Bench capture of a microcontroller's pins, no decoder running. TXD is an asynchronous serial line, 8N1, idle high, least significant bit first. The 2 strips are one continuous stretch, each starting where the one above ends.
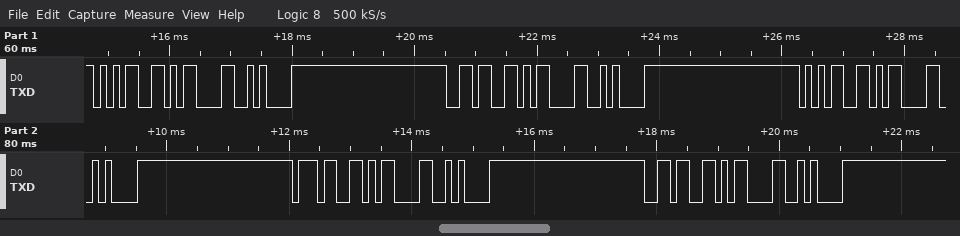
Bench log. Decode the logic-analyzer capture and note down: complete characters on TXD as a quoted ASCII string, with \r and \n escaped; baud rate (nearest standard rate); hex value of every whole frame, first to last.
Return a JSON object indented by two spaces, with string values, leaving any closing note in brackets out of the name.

{
  "complete characters on TXD as a quoted ASCII string, with \\r and \\n escaped": "\"5\\r\\n6\\r\\n5\\r\\n7\\r\\n6\\r\\n\"",
  "baud rate": "9600 baud",
  "hex value of every whole frame, first to last": "0x35 0x0D 0x0A 0x36 0x0D 0x0A 0x35 0x0D 0x0A 0x37 0x0D 0x0A 0x36 0x0D 0x0A"
}
